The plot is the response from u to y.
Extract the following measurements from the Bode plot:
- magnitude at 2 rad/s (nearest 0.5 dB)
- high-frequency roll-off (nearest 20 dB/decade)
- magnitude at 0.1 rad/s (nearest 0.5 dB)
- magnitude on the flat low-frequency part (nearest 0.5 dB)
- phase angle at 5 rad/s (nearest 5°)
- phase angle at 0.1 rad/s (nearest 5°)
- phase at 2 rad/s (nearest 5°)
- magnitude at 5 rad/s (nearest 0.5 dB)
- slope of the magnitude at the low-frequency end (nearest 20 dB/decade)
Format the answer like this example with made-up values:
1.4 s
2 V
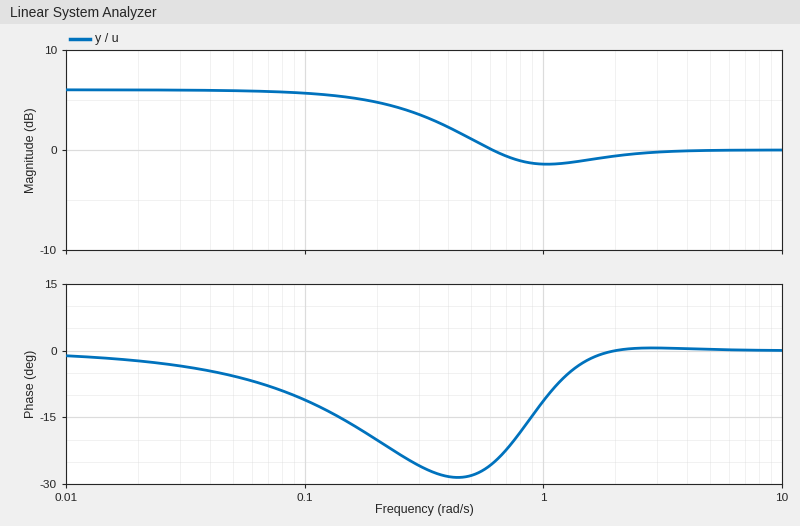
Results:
-0.5 dB
0 dB/decade
5.5 dB
6.0 dB
0°
-10°
0°
0.0 dB
0 dB/decade
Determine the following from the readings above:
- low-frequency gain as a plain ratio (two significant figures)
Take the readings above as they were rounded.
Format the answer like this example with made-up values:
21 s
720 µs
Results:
2.0
